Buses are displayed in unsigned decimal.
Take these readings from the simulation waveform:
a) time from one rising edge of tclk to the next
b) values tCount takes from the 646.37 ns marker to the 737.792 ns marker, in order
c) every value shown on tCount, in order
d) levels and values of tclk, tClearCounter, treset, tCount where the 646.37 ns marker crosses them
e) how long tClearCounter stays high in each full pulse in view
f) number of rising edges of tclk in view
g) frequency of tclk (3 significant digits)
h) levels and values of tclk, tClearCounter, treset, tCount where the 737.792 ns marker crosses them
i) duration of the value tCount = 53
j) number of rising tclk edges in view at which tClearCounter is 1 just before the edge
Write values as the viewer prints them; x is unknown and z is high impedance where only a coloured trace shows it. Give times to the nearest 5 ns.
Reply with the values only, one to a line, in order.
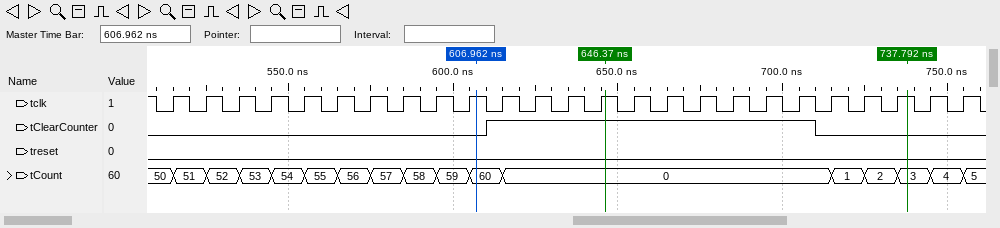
10 ns
0, 1, 2, 3
50, 51, 52, 53, 54, 55, 56, 57, 58, 59, 60, 0, 1, 2, 3, 4, 5
tclk=1, tClearCounter=1, treset=0, tCount=0
100 ns
25
100 MHz
tclk=1, tClearCounter=0, treset=0, tCount=3
10 ns
10
